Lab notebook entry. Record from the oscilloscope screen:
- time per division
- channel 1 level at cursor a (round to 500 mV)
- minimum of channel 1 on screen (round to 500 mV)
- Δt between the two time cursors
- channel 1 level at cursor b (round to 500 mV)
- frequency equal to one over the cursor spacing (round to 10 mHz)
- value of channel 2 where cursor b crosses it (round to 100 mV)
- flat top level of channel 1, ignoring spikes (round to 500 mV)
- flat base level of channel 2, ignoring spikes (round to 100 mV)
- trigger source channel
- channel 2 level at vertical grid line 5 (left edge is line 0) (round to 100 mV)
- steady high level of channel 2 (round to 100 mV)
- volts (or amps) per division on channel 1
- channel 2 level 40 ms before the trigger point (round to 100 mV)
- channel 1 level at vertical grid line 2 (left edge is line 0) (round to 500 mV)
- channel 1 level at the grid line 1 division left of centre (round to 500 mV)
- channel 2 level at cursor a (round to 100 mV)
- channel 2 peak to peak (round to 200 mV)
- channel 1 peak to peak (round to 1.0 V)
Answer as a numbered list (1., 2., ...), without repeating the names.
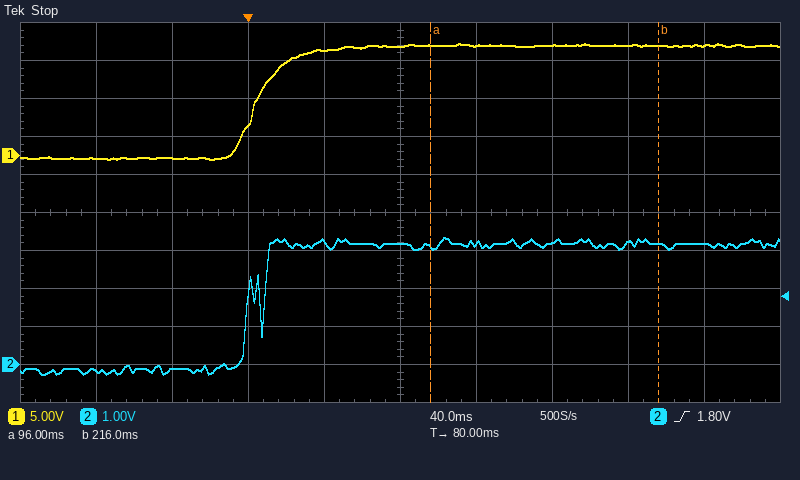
1. 40 ms
2. 14.5 V
3. -500 mV
4. 120 ms
5. 14.5 V
6. 8.33 Hz
7. 3.2 V
8. 14.5 V
9. -100 mV
10. channel 2
11. 3.2 V
12. 3.2 V
13. 5 V
14. -100 mV
15. -500 mV
16. 14.0 V
17. 3.1 V
18. 3.6 V
19. 15.0 V
